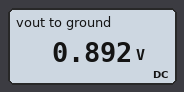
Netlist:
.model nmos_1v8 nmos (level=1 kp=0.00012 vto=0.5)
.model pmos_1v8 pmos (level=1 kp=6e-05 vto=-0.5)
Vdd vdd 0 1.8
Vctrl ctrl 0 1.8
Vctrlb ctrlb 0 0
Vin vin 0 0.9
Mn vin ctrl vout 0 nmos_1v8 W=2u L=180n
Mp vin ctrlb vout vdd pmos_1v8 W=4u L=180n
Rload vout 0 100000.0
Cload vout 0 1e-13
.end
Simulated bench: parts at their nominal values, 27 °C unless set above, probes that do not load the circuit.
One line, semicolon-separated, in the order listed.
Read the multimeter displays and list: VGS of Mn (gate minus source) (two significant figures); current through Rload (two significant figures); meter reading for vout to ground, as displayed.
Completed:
910 mV; 8.9 µA; 0.892 V
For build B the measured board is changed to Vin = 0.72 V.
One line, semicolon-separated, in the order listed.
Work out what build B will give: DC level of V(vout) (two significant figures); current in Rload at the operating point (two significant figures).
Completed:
710 mV; 7.1 µA
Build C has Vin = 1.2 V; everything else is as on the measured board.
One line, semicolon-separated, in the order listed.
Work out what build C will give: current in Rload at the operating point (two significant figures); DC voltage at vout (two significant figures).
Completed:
12 µA; 1.2 V
